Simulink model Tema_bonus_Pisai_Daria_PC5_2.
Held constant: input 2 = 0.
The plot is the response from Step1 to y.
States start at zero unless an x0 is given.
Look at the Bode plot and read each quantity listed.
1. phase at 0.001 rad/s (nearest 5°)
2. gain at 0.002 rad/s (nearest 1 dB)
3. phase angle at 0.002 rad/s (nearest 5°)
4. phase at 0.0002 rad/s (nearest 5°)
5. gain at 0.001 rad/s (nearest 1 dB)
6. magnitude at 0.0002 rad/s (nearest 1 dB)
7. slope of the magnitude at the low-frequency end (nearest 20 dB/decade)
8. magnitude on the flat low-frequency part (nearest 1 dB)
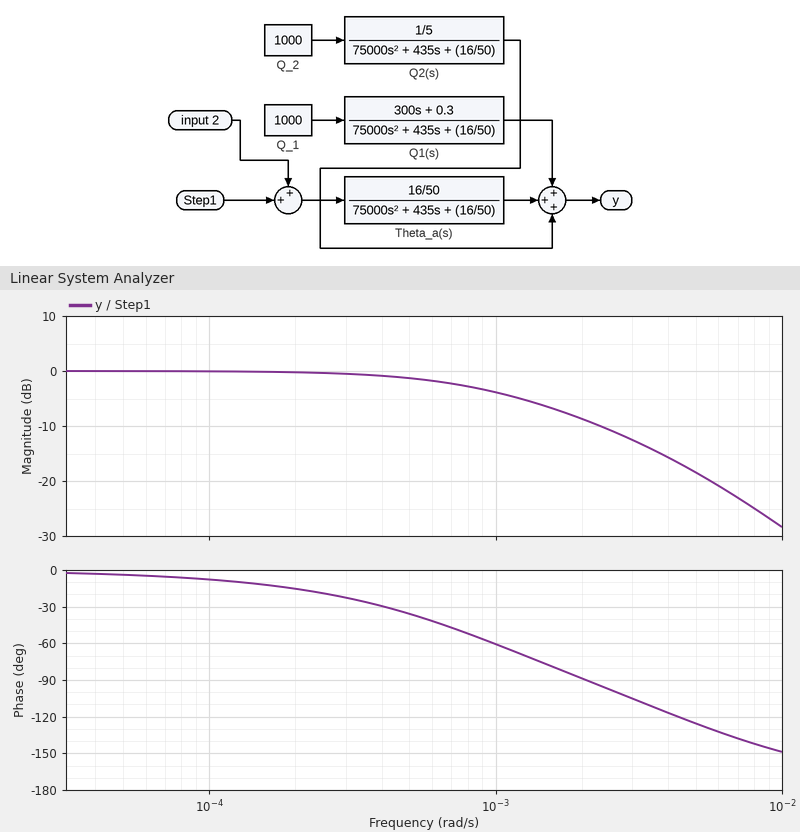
-60°
-9 dB
-90°
-15°
-4 dB
0 dB
0 dB/decade
0 dB
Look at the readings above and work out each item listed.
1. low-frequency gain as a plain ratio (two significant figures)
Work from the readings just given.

1.0
